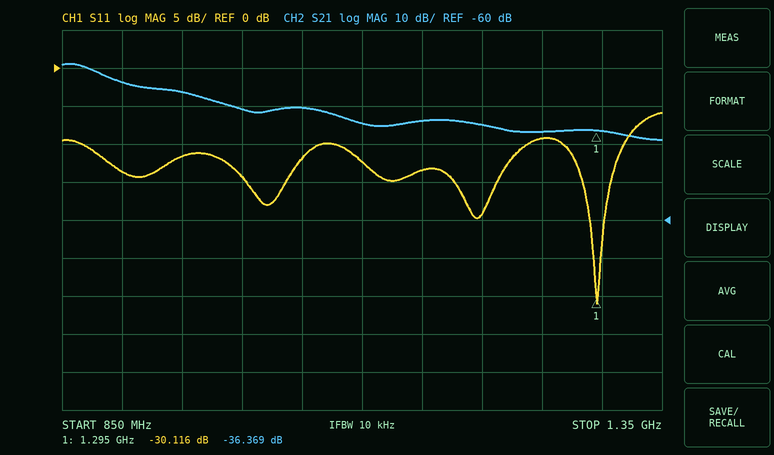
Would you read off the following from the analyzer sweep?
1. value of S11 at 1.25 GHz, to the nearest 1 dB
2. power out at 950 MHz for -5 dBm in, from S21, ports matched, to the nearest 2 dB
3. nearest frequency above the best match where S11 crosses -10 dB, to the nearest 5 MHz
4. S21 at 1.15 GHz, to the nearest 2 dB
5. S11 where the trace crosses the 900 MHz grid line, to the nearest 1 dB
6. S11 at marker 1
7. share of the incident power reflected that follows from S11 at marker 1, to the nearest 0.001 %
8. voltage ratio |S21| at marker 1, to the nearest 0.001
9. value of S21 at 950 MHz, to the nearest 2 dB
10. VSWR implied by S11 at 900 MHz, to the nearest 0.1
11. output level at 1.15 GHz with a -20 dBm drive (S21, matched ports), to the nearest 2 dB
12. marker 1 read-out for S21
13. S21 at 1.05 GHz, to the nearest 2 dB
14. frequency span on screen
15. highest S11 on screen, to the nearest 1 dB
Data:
-9 dB
-32 dBm
1.320 GHz
-34 dB
-14 dB
-30.116 dB
0.097 %
0.015
-26 dB
1.5
-54 dBm
-36.369 dB
-30 dB
500 MHz
-6 dB
